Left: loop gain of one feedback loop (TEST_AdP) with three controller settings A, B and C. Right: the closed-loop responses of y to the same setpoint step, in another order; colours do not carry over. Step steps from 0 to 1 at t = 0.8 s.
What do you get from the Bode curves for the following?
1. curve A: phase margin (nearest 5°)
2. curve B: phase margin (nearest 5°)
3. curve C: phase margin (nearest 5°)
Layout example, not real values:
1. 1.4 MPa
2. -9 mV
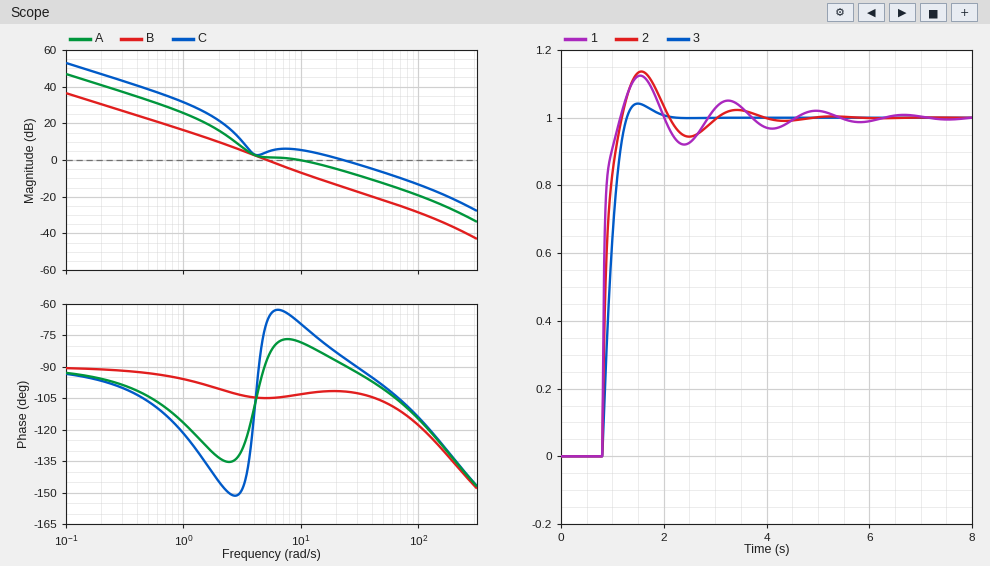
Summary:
1. 100°
2. 75°
3. 95°
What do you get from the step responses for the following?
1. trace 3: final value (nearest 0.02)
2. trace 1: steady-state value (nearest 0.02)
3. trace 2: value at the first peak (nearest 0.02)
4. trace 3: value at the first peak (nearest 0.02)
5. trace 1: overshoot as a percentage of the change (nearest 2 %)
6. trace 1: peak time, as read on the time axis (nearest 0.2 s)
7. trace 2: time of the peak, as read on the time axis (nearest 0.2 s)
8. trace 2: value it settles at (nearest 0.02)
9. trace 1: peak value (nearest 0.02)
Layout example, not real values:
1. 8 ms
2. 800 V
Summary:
1. 1.00
2. 1.00
3. 1.14
4. 1.04
5. 12 %
6. 1.6 s
7. 1.6 s
8. 1.00
9. 1.12
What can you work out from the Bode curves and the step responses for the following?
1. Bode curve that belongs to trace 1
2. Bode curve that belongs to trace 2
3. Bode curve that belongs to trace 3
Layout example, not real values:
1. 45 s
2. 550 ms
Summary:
1. C
2. A
3. B
